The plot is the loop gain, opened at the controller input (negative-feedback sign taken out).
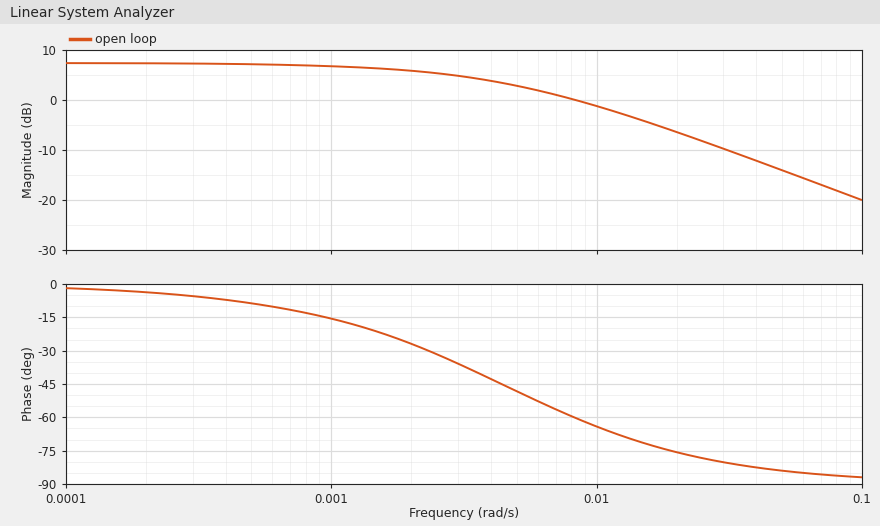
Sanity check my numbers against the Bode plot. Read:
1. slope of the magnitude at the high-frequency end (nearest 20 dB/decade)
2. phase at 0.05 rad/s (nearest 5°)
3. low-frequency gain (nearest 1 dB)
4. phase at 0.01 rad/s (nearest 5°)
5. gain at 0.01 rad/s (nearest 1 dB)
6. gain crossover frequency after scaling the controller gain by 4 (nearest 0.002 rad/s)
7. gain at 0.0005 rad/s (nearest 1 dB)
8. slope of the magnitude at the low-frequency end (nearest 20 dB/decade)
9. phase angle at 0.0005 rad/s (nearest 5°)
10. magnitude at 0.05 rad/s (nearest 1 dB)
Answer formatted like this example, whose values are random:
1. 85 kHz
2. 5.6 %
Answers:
1. -20 dB/decade
2. -85°
3. 7 dB
4. -65°
5. -1 dB
6. 0.040 rad/s
7. 7 dB
8. 0 dB/decade
9. -10°
10. -14 dB
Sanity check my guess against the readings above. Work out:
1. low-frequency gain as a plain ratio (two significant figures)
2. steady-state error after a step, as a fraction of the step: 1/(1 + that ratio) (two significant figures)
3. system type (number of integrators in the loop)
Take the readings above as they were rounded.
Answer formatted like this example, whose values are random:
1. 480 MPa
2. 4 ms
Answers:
1. 2.2
2. 0.31
3. 0
